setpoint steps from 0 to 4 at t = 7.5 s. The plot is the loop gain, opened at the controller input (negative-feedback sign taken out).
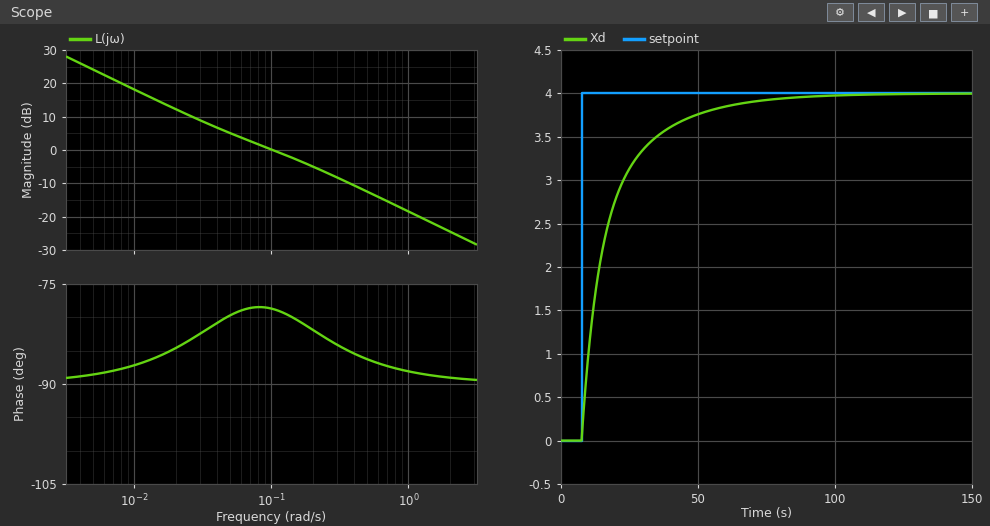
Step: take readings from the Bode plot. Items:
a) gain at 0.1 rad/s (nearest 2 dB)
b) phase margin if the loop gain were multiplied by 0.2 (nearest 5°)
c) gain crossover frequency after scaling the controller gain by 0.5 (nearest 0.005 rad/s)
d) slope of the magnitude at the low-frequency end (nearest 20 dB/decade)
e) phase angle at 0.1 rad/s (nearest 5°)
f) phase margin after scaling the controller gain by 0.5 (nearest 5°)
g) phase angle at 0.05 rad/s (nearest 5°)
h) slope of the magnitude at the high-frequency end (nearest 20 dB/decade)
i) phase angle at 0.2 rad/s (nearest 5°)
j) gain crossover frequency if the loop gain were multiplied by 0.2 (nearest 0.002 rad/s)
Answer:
0 dB
95°
0.045 rad/s
-20 dB/decade
-80°
100°
-80°
-20 dB/decade
-80°
0.016 rad/s
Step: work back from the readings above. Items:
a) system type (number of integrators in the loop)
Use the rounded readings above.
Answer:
1
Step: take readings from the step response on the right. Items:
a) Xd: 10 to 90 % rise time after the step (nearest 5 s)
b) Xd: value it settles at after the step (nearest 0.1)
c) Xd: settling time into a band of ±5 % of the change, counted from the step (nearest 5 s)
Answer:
30 s
4.0
45 s
